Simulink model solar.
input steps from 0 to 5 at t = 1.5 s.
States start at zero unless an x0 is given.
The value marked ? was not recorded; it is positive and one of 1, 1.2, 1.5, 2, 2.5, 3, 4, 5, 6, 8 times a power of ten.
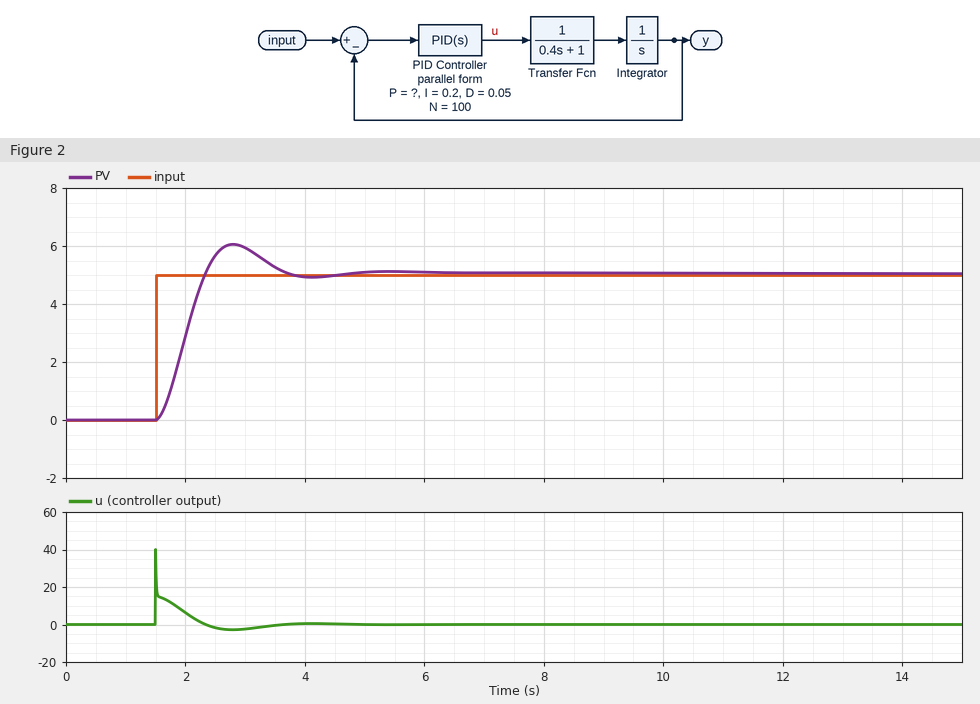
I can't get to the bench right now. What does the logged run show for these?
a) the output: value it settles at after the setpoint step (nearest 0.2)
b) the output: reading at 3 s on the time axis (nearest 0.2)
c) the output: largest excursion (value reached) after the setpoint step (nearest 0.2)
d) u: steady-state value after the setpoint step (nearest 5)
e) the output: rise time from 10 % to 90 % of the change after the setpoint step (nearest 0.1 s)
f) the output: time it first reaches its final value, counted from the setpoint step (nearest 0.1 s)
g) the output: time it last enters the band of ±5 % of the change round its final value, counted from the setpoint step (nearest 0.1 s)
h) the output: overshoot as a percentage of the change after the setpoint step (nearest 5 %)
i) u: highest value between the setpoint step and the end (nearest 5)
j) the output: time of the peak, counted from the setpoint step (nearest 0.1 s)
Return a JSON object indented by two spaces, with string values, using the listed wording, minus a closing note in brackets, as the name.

{
  "the output: value it settles at after the setpoint step": "5.0",
  "the output: reading at 3 s on the time axis": "6.0",
  "the output: largest excursion (value reached) after the setpoint step": "6.0",
  "u: steady-state value after the setpoint step": "0",
  "the output: rise time from 10 % to 90 % of the change after the setpoint step": "0.6 s",
  "the output: time it first reaches its final value, counted from the setpoint step": "0.8 s",
  "the output: time it last enters the band of ±5 % of the change round its final value, counted from the setpoint step": "2.0 s",
  "the output: overshoot as a percentage of the change after the setpoint step": "20 %",
  "u: highest value between the setpoint step and the end": "40",
  "the output: time of the peak, counted from the setpoint step": "1.3 s"
}
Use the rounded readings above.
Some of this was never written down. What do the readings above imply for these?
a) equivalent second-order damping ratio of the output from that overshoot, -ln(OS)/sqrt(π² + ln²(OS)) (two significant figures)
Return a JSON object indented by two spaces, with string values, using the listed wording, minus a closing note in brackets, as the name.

{
  "equivalent second-order damping ratio of the output from that overshoot, -ln(OS)/sqrt(π² + ln²(OS))": "0.46"
}
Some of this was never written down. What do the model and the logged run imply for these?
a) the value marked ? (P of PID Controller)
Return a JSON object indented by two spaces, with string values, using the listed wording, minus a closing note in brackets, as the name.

{
  "the value marked ?": "3"
}
